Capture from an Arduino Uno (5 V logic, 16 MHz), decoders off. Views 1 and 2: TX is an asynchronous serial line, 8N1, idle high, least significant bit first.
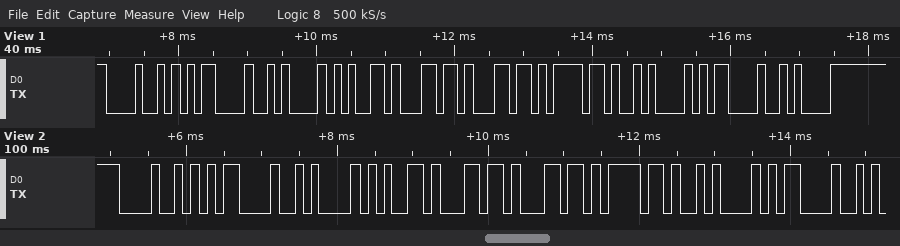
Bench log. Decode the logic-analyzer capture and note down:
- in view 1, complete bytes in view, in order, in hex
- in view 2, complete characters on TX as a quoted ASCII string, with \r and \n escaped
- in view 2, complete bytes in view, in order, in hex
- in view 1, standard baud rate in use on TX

48 0D 0A 65 6C 6C 6F 0A 0D 0A
"H\r\nello\n\r"
0x48 0x0D 0x0A 0x65 0x6C 0x6C 0x6F 0x0A 0x0D
9600 baud
